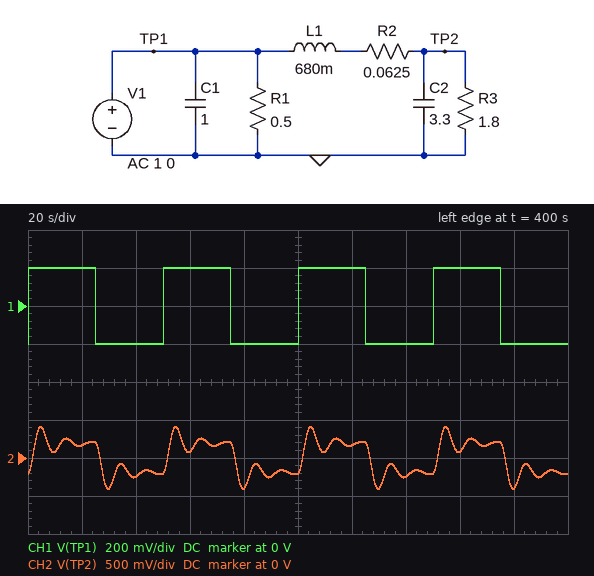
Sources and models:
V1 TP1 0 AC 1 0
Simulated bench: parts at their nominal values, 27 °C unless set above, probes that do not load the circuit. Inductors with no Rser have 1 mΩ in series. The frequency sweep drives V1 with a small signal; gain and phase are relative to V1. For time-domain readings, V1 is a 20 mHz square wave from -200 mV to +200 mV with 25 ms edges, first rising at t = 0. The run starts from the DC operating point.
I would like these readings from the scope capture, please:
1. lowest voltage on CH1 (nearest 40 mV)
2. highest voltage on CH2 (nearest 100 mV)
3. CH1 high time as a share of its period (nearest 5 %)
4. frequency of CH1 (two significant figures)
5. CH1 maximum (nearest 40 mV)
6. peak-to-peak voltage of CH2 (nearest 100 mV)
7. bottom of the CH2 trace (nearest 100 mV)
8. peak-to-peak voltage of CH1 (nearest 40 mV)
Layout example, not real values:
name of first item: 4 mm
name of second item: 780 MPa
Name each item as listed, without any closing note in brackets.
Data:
lowest voltage on CH1: -200 mV
highest voltage on CH2: 400 mV
CH1 high time as a share of its period: 50 %
frequency of CH1: 20 mHz
CH1 maximum: 200 mV
peak-to-peak voltage of CH2: 800 mV
bottom of the CH2 trace: -400 mV
peak-to-peak voltage of CH1: 400 mV
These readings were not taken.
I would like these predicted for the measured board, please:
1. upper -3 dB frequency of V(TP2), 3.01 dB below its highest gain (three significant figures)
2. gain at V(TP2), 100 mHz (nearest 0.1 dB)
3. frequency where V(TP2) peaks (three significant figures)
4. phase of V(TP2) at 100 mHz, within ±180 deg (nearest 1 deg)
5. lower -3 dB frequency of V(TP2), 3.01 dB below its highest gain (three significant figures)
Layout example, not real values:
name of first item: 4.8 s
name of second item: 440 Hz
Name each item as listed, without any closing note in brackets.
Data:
upper -3 dB frequency of V(TP2), 3.01 dB below its highest gain: 123 mHz
gain at V(TP2), 100 mHz: 8.0 dB
frequency where V(TP2) peaks: 104 mHz
phase of V(TP2) at 100 mHz, within ±180 deg: -68 deg
lower -3 dB frequency of V(TP2), 3.01 dB below its highest gain: 80.0 mHz
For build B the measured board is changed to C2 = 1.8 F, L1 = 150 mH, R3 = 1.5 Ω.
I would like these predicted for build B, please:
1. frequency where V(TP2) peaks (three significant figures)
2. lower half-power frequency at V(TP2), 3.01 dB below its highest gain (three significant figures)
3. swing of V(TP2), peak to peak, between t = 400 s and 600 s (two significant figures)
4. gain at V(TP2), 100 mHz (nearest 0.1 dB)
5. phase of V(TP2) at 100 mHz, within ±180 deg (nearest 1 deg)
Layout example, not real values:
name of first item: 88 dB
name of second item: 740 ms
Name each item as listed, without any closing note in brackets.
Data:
frequency where V(TP2) peaks: 300 mHz
lower half-power frequency at V(TP2), 3.01 dB below its highest gain: 226 mHz
swing of V(TP2), peak to peak, between t = 400 s and 600 s: 790 mV
gain at V(TP2), 100 mHz: 0.5 dB
phase of V(TP2) at 100 mHz, within ±180 deg: -8 deg
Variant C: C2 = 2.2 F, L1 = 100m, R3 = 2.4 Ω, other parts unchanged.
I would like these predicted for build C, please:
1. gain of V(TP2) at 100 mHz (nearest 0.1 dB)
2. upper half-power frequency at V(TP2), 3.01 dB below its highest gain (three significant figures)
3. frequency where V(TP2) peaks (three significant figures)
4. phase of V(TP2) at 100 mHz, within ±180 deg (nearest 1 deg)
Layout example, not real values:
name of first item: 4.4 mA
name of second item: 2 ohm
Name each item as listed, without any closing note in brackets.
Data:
gain of V(TP2) at 100 mHz: 0.5 dB
upper half-power frequency at V(TP2), 3.01 dB below its highest gain: 392 mHz
frequency where V(TP2) peaks: 331 mHz
phase of V(TP2) at 100 mHz, within ±180 deg: -7 deg
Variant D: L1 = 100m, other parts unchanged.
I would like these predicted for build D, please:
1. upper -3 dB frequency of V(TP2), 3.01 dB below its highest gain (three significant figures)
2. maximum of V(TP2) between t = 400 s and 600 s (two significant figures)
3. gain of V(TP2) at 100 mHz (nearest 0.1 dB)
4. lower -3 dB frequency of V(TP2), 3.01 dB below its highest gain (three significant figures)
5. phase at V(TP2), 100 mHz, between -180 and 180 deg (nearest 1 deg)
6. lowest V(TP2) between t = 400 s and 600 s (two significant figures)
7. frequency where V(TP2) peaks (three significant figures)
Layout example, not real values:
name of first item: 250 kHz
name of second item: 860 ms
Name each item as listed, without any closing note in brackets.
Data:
upper -3 dB frequency of V(TP2), 3.01 dB below its highest gain: 326 mHz
maximum of V(TP2) between t = 400 s and 600 s: 380 mV
gain of V(TP2) at 100 mHz: 0.7 dB
lower -3 dB frequency of V(TP2), 3.01 dB below its highest gain: 190 mHz
phase at V(TP2), 100 mHz, between -180 and 180 deg: -10 deg
lowest V(TP2) between t = 400 s and 600 s: -380 mV
frequency where V(TP2) peaks: 267 mHz
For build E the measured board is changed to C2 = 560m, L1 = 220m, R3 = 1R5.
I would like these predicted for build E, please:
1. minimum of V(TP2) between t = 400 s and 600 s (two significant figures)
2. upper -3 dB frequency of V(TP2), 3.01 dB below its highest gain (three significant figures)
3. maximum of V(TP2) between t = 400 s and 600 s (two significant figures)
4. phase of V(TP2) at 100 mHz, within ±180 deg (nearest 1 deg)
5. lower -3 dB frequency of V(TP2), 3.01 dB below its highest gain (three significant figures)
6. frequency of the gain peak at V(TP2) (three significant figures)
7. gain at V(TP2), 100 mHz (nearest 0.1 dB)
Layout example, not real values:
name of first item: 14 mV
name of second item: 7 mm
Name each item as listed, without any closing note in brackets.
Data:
minimum of V(TP2) between t = 400 s and 600 s: -360 mV
upper -3 dB frequency of V(TP2), 3.01 dB below its highest gain: 540 mHz
maximum of V(TP2) between t = 400 s and 600 s: 360 mV
phase of V(TP2) at 100 mHz, within ±180 deg: -7 deg
lower -3 dB frequency of V(TP2), 3.01 dB below its highest gain: 285 mHz
frequency of the gain peak at V(TP2): 432 mHz
gain at V(TP2), 100 mHz: 0 dB
